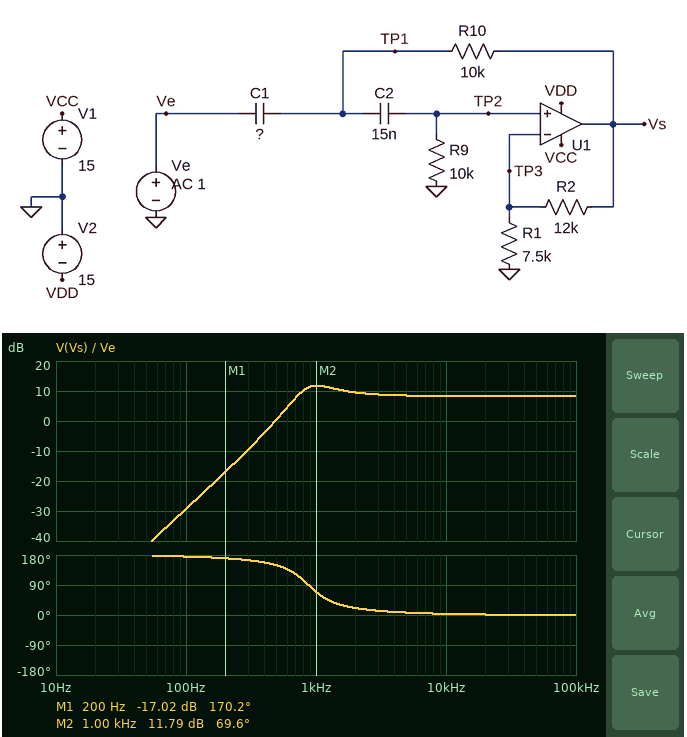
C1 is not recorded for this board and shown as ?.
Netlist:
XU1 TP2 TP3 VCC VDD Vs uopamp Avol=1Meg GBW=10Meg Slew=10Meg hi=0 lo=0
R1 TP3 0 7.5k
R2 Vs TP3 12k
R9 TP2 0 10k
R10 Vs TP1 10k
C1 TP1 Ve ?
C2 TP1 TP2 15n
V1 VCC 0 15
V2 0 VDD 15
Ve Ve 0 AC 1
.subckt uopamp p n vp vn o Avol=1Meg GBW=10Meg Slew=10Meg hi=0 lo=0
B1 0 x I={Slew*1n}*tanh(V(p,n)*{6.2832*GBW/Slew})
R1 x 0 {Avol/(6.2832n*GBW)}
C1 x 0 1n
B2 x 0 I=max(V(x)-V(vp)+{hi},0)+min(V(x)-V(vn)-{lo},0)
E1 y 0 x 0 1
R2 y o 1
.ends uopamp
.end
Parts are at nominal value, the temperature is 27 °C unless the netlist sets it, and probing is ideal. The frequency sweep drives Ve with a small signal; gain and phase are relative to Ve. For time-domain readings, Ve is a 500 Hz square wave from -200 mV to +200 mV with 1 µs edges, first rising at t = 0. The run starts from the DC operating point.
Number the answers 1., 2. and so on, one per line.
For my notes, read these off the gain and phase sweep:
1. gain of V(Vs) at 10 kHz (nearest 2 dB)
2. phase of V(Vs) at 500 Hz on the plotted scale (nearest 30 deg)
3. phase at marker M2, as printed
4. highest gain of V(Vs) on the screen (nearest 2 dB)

1. 8 dB
2. 150 deg
3. 69.6 deg
4. 12 dB
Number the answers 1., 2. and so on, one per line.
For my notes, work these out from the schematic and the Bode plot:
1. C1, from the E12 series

1. 22 nF
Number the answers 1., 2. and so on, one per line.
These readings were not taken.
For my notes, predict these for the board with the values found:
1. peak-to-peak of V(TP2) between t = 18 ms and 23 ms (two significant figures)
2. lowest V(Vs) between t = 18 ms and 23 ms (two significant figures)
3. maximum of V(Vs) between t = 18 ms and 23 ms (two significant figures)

1. 710 mV
2. -920 mV
3. 920 mV
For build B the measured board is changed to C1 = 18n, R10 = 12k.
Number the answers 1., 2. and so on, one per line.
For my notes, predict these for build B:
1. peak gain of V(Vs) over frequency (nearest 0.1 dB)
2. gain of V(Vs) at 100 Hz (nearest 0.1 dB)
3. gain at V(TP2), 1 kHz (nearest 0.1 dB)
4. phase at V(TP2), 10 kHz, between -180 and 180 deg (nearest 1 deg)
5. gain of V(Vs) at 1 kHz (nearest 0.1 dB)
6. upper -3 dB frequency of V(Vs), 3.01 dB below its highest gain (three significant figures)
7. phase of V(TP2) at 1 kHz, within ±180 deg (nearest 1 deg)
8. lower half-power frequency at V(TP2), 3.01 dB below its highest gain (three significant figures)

1. 10.4 dB
2. -29.5 dB
3. 2.0 dB
4. 4 deg
5. 10.3 dB
6. 1.80 MHz
7. 74 deg
8. 746 Hz
